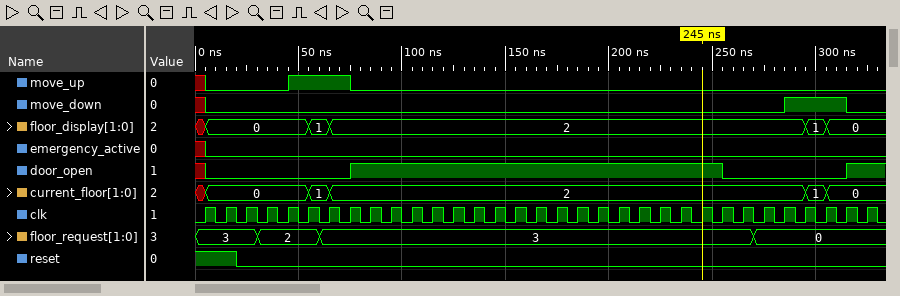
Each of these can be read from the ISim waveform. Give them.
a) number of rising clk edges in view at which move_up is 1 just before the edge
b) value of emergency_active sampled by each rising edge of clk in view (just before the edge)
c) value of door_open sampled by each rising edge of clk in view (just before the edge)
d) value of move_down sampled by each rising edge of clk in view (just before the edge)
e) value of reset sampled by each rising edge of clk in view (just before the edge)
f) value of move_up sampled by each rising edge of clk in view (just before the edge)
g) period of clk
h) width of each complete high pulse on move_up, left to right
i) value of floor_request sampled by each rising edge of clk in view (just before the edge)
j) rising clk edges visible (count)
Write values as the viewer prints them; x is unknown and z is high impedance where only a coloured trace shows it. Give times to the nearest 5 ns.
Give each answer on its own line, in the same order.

3
x 0 0 0 0 0 0 0 0 0 0 0 0 0 0 0 0 0 0 0 0 0 0 0 0 0 0 0 0 0 0 0 0
x 0 0 0 0 0 0 0 1 1 1 1 1 1 1 1 1 1 1 1 1 1 1 1 1 1 0 0 0 0 0 0 1
x 0 0 0 0 0 0 0 0 0 0 0 0 0 0 0 0 0 0 0 0 0 0 0 0 0 0 0 0 1 1 1 0
1 1 0 0 0 0 0 0 0 0 0 0 0 0 0 0 0 0 0 0 0 0 0 0 0 0 0 0 0 0 0 0 0
x 0 0 0 0 1 1 1 0 0 0 0 0 0 0 0 0 0 0 0 0 0 0 0 0 0 0 0 0 0 0 0 0
10 ns
30 ns
3, 3, 3, 2, 2, 2, 3, 3, 3, 3, 3, 3, 3, 3, 3, 3, 3, 3, 3, 3, 3, 3, 3, 3, 3, 3, 3, 0, 0, 0, 0, 0, 0
33
